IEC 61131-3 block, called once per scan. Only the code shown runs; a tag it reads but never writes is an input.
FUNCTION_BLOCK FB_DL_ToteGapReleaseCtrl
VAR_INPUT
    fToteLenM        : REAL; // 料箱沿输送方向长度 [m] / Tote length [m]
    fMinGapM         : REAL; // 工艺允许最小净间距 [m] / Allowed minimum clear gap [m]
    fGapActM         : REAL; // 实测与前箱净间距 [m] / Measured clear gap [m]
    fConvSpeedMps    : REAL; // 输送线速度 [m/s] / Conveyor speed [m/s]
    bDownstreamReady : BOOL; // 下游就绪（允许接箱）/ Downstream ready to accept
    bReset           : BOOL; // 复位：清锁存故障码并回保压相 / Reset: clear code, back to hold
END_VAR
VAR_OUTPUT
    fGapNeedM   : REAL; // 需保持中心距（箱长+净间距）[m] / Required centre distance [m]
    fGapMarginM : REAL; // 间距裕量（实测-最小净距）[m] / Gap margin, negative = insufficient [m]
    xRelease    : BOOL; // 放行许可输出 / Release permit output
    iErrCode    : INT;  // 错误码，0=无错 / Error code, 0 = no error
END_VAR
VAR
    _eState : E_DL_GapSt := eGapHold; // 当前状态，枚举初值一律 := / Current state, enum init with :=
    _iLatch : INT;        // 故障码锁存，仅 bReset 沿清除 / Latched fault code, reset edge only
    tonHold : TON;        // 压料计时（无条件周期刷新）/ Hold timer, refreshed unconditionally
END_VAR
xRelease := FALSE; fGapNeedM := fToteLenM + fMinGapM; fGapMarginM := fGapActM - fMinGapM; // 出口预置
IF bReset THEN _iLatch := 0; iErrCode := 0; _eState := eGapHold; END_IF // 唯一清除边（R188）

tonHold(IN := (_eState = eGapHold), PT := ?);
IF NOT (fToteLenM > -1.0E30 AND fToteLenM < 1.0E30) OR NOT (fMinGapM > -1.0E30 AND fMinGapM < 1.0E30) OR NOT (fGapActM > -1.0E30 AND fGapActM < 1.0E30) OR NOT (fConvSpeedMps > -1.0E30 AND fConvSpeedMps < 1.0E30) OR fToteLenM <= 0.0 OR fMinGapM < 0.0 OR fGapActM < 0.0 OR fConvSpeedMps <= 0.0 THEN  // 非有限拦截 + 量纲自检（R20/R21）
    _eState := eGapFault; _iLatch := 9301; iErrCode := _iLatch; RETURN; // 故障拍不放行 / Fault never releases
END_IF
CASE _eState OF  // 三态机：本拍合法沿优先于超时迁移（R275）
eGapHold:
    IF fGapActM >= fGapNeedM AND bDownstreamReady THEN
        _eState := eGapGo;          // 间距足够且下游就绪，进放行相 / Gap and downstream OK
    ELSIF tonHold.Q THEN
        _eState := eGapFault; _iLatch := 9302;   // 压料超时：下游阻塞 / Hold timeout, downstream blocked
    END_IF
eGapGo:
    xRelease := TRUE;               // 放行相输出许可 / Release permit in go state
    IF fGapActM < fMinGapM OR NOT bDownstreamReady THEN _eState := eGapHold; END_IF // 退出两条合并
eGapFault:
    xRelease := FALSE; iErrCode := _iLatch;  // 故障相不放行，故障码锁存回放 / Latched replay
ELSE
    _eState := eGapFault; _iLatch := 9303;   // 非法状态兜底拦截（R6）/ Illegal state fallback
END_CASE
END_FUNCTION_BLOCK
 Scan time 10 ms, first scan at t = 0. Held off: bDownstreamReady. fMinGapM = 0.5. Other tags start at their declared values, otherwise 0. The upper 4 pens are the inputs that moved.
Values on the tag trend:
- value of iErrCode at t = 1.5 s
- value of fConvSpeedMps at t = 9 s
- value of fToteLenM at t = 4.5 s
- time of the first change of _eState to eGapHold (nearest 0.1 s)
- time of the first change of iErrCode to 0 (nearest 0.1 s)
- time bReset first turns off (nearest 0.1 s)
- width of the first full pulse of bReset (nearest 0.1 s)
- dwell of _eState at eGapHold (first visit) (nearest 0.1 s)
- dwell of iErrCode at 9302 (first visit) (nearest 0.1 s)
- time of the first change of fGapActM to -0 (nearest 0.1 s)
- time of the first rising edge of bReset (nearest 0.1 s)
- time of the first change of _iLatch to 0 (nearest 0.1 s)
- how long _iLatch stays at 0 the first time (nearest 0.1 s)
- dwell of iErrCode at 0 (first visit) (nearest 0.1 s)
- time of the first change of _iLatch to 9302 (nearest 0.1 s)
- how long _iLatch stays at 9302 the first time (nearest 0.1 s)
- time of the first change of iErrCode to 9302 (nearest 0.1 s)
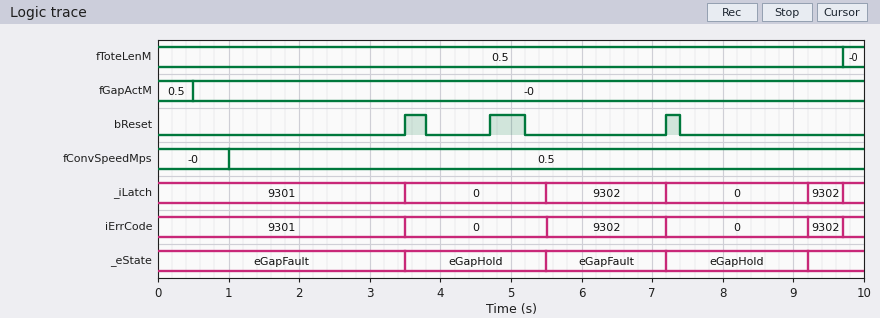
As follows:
9301
0.5
0.5
3.5 s
3.5 s
3.8 s
0.3 s
2.0 s
1.7 s
0.5 s
3.5 s
3.5 s
2.0 s
2.0 s
5.5 s
1.7 s
5.5 s
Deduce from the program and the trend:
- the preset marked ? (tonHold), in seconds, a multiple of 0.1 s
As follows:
2.0 s
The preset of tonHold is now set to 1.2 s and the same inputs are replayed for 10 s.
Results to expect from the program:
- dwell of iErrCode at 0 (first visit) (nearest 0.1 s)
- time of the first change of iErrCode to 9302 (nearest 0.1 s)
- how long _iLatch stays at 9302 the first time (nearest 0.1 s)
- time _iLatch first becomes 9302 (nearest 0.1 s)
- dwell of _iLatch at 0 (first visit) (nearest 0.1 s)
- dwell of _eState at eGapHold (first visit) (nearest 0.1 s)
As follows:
1.7 s
5.2 s
2.5 s
4.7 s
1.2 s
1.2 s
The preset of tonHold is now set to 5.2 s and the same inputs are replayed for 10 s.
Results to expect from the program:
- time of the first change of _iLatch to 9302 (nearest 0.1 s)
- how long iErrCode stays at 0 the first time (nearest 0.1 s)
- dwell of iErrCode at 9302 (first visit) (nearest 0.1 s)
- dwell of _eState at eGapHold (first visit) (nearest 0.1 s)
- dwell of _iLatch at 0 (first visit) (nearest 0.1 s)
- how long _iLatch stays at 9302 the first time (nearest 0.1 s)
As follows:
8.7 s
5.2 s
1.0 s
5.2 s
5.2 s
1.0 s
